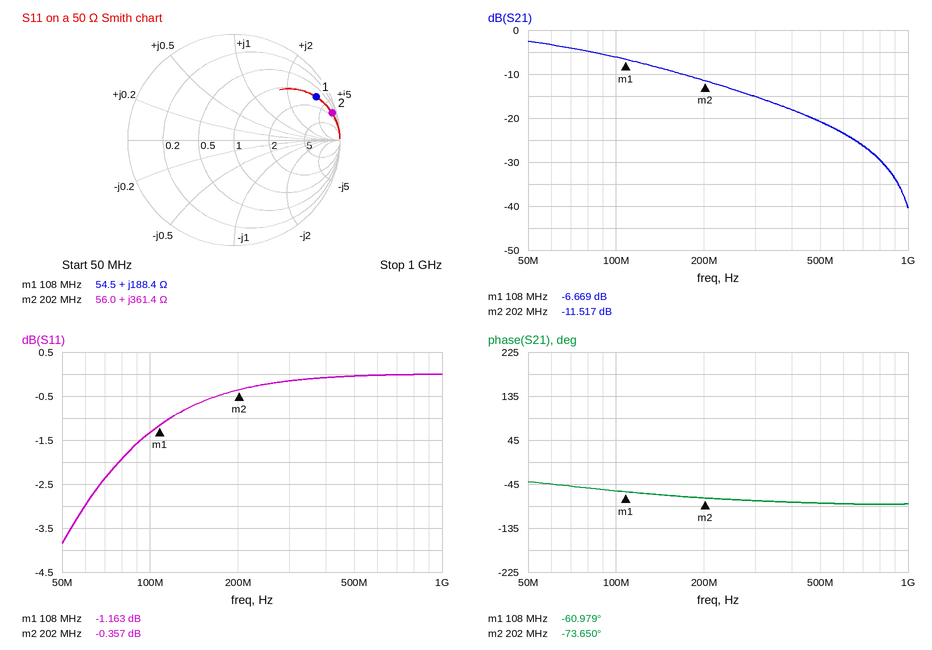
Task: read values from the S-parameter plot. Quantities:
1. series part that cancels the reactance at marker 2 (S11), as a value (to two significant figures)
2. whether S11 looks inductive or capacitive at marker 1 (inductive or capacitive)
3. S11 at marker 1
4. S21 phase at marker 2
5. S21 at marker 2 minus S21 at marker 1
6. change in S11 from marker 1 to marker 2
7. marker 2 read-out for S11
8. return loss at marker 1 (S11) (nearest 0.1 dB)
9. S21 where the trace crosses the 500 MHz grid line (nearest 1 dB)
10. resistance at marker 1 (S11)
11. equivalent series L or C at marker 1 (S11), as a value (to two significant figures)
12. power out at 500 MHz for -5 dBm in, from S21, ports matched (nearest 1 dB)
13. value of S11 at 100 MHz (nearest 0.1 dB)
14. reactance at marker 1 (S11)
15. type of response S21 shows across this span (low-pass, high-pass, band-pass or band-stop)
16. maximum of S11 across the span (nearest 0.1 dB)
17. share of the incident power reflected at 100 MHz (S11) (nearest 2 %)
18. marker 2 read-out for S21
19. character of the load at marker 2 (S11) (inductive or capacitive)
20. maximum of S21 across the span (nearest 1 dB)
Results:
2.2 pF
inductive
-1.163 dB
-73.650°
-4.848 dB
0.806 dB
-0.357 dB
1.2 dB
-21 dB
54.5 Ω
280 nH
-26 dBm
-1.3 dB
+188.4 Ω
low-pass
0.0 dB
74 %
-11.517 dB
inductive
-3 dB
